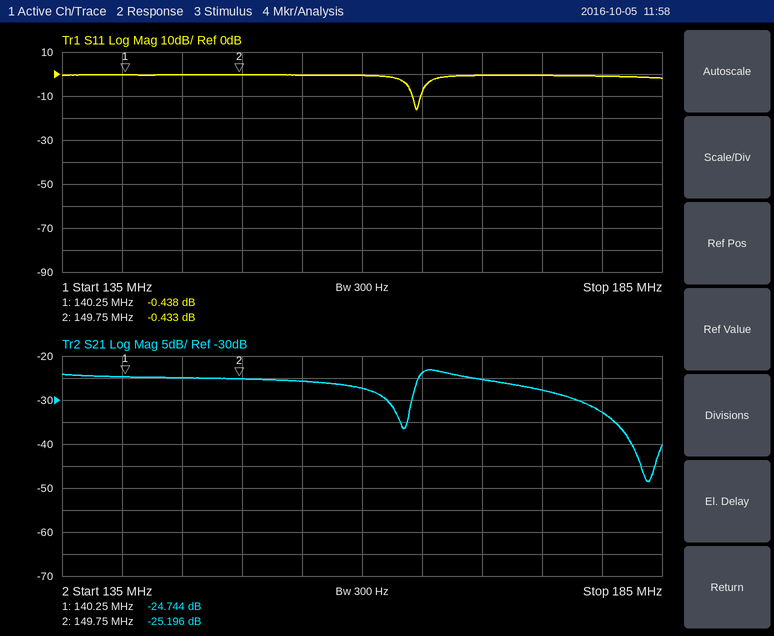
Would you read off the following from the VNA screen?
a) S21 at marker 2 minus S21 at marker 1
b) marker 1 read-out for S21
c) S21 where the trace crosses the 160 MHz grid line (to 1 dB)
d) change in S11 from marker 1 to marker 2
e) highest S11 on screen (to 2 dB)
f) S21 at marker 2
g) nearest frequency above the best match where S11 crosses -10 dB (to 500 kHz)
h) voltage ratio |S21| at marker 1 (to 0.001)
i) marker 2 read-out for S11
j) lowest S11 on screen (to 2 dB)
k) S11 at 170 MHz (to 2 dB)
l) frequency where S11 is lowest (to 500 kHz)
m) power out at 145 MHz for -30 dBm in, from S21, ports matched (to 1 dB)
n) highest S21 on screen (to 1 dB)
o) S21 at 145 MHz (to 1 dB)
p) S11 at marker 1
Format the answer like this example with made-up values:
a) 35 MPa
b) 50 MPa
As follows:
a) -0.452 dB
b) -24.744 dB
c) -27 dB
d) 0.005 dB
e) 0 dB
f) -25.196 dB
g) 165.0 MHz
h) 0.058
i) -0.433 dB
j) -16 dB
k) 0 dB
l) 164.5 MHz
m) -55 dBm
n) -23 dB
o) -25 dB
p) -0.438 dB
